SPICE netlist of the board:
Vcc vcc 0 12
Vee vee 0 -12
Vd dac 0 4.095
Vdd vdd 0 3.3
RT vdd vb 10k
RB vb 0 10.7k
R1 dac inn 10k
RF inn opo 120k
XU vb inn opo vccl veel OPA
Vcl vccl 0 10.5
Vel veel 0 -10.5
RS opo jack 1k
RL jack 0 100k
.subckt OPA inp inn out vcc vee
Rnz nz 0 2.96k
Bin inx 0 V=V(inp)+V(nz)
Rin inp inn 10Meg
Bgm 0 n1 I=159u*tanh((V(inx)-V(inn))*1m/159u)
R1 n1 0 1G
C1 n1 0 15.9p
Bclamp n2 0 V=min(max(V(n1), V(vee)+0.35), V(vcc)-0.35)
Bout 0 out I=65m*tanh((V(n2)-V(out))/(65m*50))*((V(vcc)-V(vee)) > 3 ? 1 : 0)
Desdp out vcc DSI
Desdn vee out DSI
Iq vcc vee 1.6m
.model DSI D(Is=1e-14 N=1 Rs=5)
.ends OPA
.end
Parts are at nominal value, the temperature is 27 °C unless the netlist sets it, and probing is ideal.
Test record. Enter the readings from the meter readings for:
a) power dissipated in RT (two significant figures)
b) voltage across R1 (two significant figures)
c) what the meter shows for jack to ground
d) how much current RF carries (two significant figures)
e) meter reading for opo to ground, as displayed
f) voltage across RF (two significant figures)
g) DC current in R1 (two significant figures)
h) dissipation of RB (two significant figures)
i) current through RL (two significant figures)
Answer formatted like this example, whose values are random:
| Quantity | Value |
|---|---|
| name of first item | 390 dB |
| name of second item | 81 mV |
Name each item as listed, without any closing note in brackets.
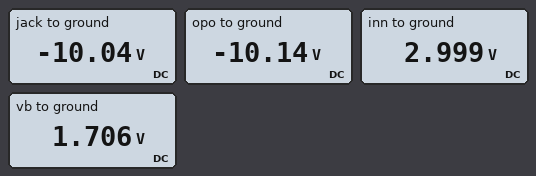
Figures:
| Quantity | Value |
|---|---|
| power dissipated in RT | 250 µW |
| voltage across R1 | 1.1 V |
| what the meter shows for jack to ground | -10.04 V |
| how much current RF carries | 110 µA |
| meter reading for opo to ground, as displayed | -10.14 V |
| voltage across RF | 13 V |
| DC current in R1 | 110 µA |
| dissipation of RB | 270 µW |
| current through RL | 100 µA |
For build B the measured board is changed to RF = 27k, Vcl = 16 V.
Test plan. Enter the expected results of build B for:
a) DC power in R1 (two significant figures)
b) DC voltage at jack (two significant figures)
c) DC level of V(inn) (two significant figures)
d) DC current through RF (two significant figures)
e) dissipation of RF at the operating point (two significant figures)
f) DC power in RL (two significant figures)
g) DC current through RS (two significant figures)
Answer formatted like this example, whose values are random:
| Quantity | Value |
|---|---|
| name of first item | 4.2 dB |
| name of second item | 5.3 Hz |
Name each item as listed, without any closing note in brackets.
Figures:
| Quantity | Value |
|---|---|
| DC power in R1 | 570 µW |
| DC voltage at jack | -4.7 V |
| DC level of V(inn) | 1.7 V |
| DC current through RF | 240 µA |
| dissipation of RF at the operating point | 1.5 mW |
| DC power in RL | 220 µW |
| DC current through RS | 47 µA |
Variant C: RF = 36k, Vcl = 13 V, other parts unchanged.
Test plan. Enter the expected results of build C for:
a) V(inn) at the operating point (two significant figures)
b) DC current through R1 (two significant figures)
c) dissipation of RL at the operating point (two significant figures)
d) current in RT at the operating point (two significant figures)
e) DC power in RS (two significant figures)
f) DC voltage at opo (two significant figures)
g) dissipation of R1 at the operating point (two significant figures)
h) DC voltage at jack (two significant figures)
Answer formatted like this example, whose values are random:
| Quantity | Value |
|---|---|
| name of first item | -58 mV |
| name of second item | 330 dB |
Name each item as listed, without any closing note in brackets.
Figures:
| Quantity | Value |
|---|---|
| V(inn) at the operating point | 1.7 V |
| DC current through R1 | 240 µA |
| dissipation of RL at the operating point | 470 µW |
| current in RT at the operating point | 160 µA |
| DC power in RS | 4.7 µW |
| DC voltage at opo | -6.9 V |
| dissipation of R1 at the operating point | 570 µW |
| DC voltage at jack | -6.8 V |
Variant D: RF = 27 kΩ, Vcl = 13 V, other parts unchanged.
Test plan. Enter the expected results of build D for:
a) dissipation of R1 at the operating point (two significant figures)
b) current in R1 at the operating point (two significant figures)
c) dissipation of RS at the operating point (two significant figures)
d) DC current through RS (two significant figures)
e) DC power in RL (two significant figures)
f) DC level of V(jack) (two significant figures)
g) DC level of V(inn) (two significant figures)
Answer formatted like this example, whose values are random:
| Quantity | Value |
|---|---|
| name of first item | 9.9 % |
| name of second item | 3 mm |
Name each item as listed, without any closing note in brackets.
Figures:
| Quantity | Value |
|---|---|
| dissipation of R1 at the operating point | 570 µW |
| current in R1 at the operating point | 240 µA |
| dissipation of RS at the operating point | 2.2 µW |
| DC current through RS | 47 µA |
| DC power in RL | 220 µW |
| DC level of V(jack) | -4.7 V |
| DC level of V(inn) | 1.7 V |
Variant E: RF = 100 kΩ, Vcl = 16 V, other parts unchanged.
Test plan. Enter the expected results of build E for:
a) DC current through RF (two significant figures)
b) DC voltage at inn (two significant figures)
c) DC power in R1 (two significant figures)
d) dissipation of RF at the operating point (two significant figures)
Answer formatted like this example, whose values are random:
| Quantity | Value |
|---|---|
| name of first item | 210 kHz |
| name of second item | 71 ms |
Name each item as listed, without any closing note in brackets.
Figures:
| Quantity | Value |
|---|---|
| DC current through RF | 130 µA |
| DC voltage at inn | 2.8 V |
| DC power in R1 | 170 µW |
| dissipation of RF at the operating point | 1.7 mW |
